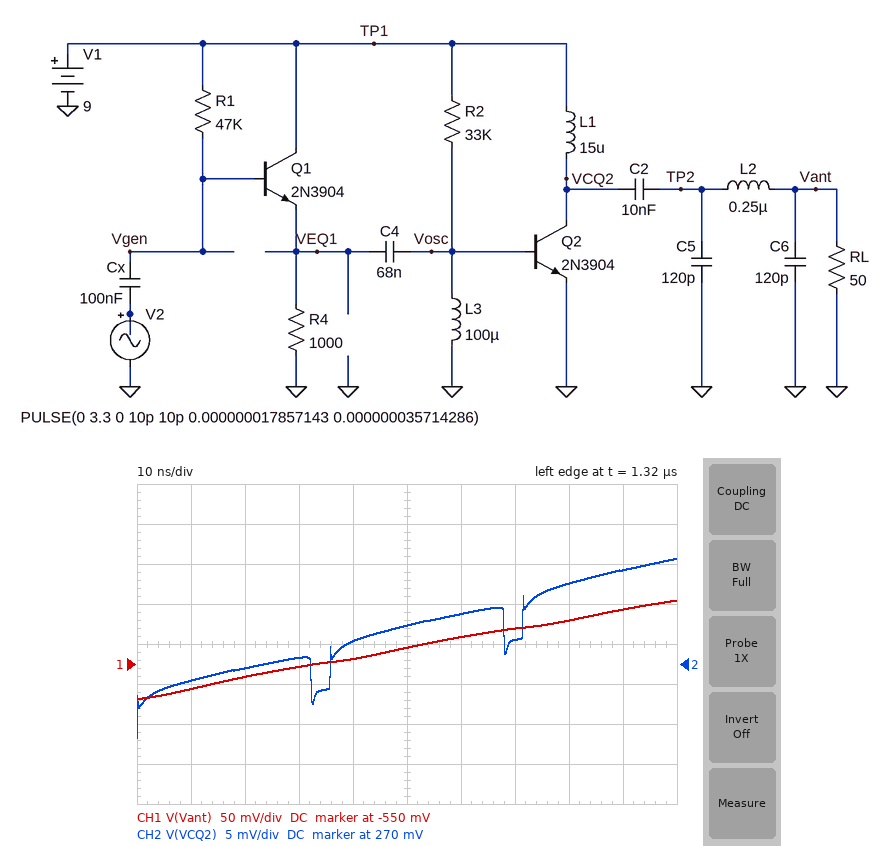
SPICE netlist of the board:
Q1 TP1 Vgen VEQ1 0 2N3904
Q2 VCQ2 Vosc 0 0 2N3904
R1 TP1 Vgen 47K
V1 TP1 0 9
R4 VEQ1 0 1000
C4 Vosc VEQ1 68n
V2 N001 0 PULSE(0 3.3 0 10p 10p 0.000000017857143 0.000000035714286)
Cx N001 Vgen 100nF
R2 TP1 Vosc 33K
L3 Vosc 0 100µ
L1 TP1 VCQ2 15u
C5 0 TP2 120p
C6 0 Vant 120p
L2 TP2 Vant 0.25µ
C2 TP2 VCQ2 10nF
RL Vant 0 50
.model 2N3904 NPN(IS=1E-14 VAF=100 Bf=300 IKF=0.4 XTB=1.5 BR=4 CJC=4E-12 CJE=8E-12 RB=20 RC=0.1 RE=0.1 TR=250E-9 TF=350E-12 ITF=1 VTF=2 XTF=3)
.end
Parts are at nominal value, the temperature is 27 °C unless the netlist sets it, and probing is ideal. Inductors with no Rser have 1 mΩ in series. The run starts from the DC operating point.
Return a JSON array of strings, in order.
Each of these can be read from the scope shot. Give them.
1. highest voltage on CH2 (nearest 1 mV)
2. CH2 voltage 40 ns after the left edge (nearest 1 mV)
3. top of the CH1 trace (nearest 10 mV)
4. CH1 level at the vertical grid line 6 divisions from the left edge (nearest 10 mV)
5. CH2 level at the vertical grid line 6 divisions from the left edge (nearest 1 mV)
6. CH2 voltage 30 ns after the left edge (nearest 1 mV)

["283 mV", "273 mV", "-470 mV", "-520 mV", "276 mV", "271 mV"]
